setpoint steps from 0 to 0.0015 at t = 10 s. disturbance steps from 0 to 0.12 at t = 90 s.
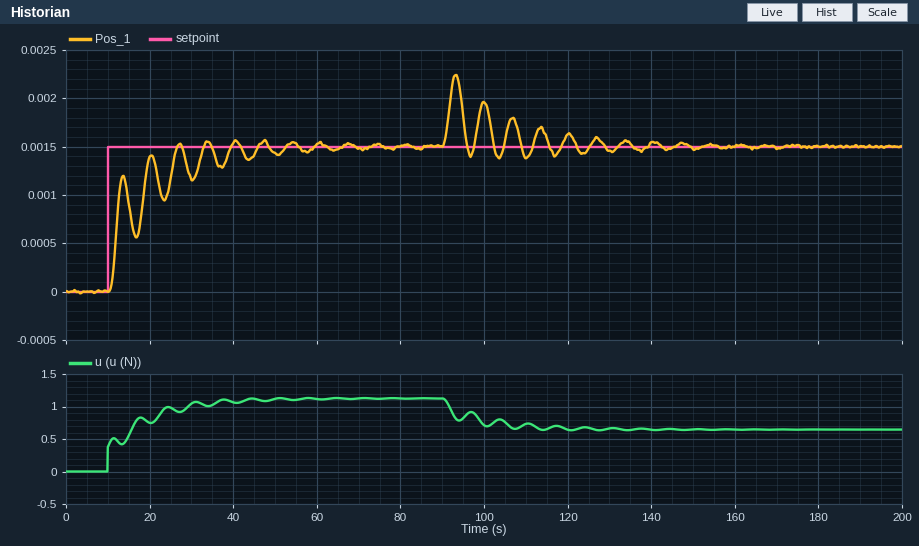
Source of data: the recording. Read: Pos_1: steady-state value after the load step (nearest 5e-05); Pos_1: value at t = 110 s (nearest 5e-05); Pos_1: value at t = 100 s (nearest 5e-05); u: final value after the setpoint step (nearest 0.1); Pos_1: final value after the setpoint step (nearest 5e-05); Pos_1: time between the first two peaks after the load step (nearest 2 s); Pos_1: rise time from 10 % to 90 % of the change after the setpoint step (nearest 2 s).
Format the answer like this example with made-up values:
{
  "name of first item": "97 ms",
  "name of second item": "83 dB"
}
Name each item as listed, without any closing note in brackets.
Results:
{
  "Pos_1: steady-state value after the load step": "0.00150",
  "Pos_1: value at t = 110 s": "0.00140",
  "Pos_1: value at t = 100 s": "0.00195",
  "u: final value after the setpoint step": "1.1",
  "Pos_1: final value after the setpoint step": "0.00150",
  "Pos_1: time between the first two peaks after the load step": "6 s",
  "Pos_1: rise time from 10 % to 90 % of the change after the setpoint step": "8 s"
}
